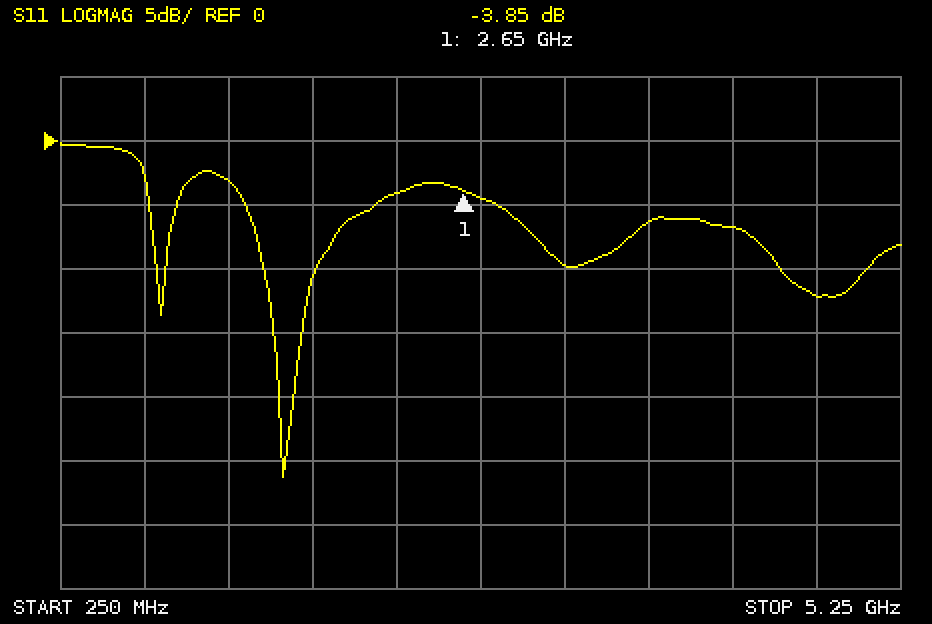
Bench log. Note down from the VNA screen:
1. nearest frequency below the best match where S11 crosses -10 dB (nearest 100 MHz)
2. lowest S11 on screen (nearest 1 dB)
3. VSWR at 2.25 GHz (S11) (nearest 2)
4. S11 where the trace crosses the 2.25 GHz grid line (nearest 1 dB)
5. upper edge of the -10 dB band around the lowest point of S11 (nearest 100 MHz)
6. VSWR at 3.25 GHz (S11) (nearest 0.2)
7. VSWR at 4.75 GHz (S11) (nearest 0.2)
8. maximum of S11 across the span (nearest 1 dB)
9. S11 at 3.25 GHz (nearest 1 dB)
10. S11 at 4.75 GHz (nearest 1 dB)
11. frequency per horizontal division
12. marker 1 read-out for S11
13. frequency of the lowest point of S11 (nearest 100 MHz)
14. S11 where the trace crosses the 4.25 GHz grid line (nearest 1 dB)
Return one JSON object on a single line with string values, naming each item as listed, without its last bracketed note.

{"nearest frequency below the best match where S11 crosses -10 dB": "1.5 GHz", "lowest S11 on screen": "-26 dB", "VSWR at 2.25 GHz (S11)": "4", "S11 where the trace crosses the 2.25 GHz grid line": "-4 dB", "upper edge of the -10 dB band around the lowest point of S11": "1.8 GHz", "VSWR at 3.25 GHz (S11)": "2.0", "VSWR at 4.75 GHz (S11)": "1.6", "maximum of S11 across the span": "0 dB", "S11 at 3.25 GHz": "-10 dB", "S11 at 4.75 GHz": "-12 dB", "frequency per horizontal division": "500 MHz", "marker 1 read-out for S11": "-3.85 dB", "frequency of the lowest point of S11": "1.6 GHz", "S11 where the trace crosses the 4.25 GHz grid line": "-7 dB"}
